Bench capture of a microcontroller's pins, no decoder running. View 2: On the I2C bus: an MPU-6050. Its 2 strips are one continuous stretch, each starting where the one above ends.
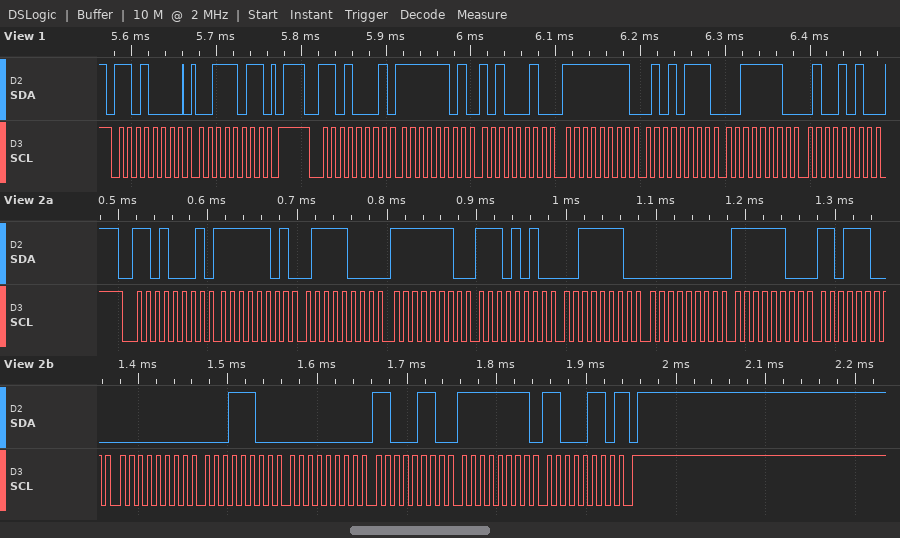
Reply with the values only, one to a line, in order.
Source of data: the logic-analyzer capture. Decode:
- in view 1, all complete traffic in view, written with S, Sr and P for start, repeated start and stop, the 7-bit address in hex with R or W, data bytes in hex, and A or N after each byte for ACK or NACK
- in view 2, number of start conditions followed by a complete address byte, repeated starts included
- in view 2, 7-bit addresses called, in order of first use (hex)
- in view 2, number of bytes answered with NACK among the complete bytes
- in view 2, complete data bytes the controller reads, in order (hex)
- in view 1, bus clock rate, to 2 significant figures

S 68W A 3B A P S 68R A FD A A2 A FF A 57 A 3E A 4A A
1
0x68
1
FD 78 FE EA 3E 00 FC DC 00 1C 00 C6 FF C6
100 kHz
